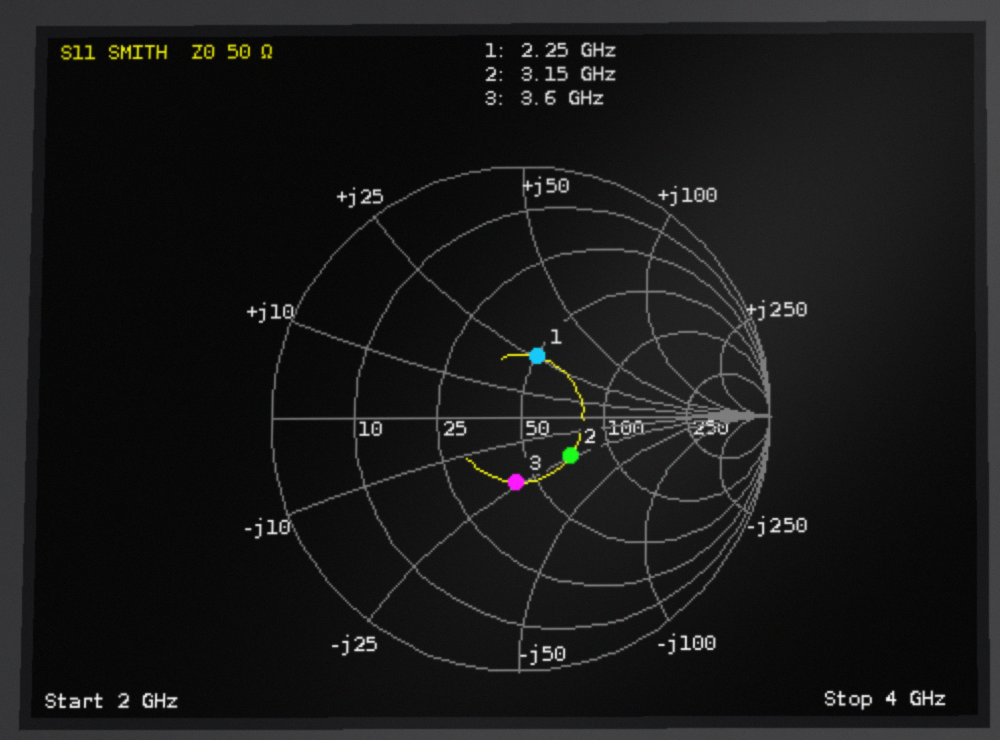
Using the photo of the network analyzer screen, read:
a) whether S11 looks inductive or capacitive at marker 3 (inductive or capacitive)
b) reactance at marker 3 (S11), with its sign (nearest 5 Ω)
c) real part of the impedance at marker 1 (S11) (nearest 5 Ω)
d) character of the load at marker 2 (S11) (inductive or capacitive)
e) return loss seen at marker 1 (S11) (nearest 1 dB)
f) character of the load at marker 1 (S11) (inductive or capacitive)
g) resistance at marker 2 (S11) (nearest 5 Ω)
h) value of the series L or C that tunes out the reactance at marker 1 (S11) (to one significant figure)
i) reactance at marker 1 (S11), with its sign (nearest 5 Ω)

capacitive
-25 Ω
50 Ω
capacitive
12 dB
inductive
70 Ω
3 pF
+25 Ω
